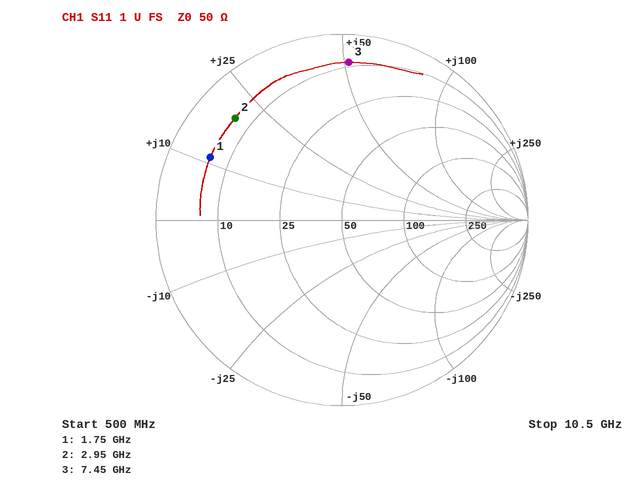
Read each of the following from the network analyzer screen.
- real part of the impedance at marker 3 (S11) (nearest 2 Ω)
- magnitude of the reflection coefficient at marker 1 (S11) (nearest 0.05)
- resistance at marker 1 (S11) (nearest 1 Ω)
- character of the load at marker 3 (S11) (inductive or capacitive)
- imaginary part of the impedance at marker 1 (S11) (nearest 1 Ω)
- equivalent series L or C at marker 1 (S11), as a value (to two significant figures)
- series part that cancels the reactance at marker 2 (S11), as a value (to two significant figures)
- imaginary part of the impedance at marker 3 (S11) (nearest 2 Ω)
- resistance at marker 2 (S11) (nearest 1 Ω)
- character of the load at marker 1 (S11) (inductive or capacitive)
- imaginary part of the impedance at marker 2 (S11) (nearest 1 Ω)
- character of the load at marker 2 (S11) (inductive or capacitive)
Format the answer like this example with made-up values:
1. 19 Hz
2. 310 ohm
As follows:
1. 8 Ω
2. 0.80
3. 6 Ω
4. inductive
5. +11 Ω
6. 1.0 nH
7. 2.7 pF
8. +52 Ω
9. 7 Ω
10. inductive
11. +20 Ω
12. inductive
